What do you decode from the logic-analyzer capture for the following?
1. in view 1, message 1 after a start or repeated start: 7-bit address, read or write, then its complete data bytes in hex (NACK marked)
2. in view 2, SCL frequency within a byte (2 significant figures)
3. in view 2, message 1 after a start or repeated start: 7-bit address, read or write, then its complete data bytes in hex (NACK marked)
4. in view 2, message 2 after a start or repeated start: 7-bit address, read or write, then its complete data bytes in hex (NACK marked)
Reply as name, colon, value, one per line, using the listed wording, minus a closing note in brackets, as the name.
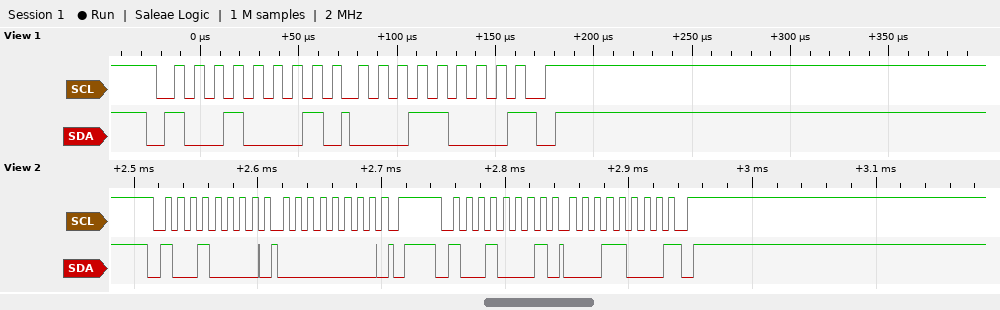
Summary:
in view 1, message 1 after a start or repeated start: 7-bit address, read or write, then its complete data bytes in hex: 0x48 read: 18 NACK
in view 2, SCL frequency within a byte: 100 kHz
in view 2, message 1 after a start or repeated start: 7-bit address, read or write, then its complete data bytes in hex: 0x48 write: 00
in view 2, message 2 after a start or repeated start: 7-bit address, read or write, then its complete data bytes in hex: 0x48 read: 18 NACK
